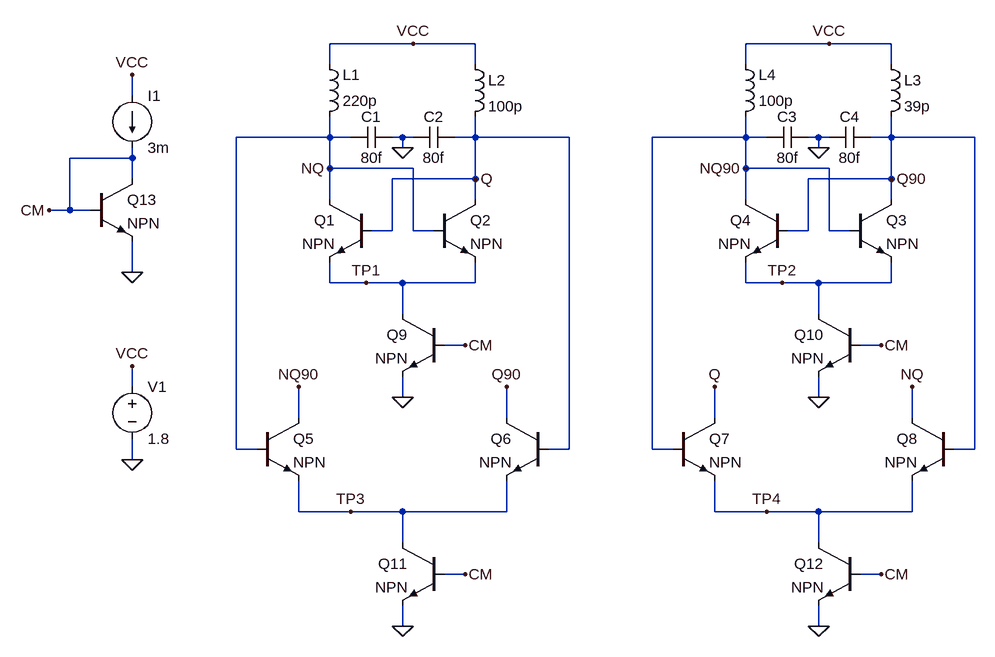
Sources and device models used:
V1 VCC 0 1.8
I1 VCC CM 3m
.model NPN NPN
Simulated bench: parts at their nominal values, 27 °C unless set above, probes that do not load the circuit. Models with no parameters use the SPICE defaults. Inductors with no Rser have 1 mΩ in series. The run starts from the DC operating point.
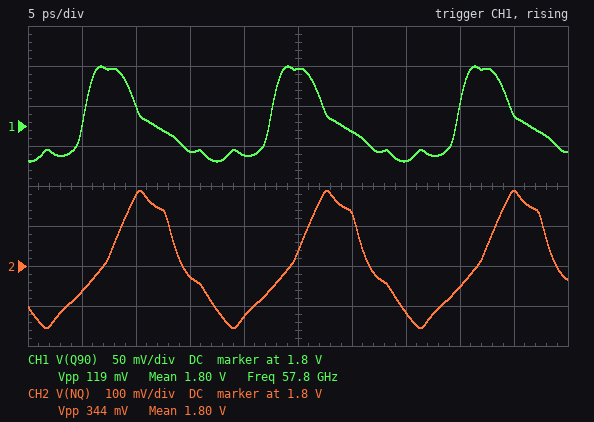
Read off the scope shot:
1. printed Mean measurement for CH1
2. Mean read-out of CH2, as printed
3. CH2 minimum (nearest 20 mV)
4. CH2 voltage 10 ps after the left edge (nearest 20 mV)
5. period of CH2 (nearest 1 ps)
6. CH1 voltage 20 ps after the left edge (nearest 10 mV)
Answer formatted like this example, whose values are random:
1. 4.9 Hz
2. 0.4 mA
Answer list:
1. 1.80 V
2. 1.80 V
3. 1.64 V
4. 1.98 V
5. 17 ps
6. 1.76 V
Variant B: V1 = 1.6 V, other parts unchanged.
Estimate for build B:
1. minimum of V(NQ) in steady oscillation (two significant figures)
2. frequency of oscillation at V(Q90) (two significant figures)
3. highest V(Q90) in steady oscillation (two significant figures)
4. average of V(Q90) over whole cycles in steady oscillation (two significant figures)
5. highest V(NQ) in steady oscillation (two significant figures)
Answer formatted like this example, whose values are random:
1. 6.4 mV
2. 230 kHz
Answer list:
1. 1.4 V
2. 58 GHz
3. 1.7 V
4. 1.6 V
5. 1.8 V
